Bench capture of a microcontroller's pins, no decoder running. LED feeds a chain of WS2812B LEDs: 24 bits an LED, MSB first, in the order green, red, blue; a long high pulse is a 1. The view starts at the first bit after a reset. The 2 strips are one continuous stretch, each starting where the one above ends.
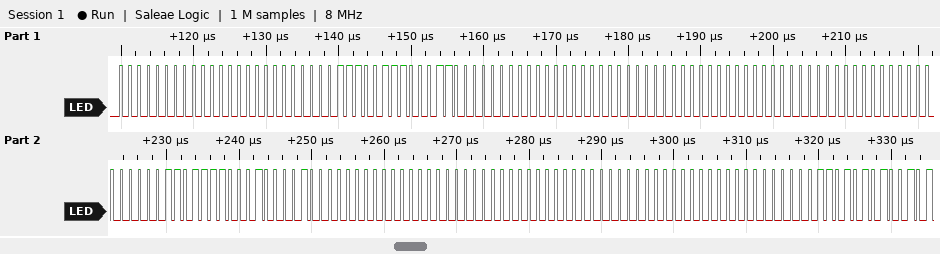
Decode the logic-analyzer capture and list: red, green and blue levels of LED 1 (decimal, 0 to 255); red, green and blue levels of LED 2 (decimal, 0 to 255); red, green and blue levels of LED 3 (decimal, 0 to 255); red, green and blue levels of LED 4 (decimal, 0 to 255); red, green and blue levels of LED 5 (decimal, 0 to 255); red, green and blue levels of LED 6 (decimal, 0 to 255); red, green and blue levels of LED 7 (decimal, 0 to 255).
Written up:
0, 0, 0
24, 231, 0
0, 0, 0
0, 0, 0
33, 222, 0
0, 0, 0
0, 0, 0
